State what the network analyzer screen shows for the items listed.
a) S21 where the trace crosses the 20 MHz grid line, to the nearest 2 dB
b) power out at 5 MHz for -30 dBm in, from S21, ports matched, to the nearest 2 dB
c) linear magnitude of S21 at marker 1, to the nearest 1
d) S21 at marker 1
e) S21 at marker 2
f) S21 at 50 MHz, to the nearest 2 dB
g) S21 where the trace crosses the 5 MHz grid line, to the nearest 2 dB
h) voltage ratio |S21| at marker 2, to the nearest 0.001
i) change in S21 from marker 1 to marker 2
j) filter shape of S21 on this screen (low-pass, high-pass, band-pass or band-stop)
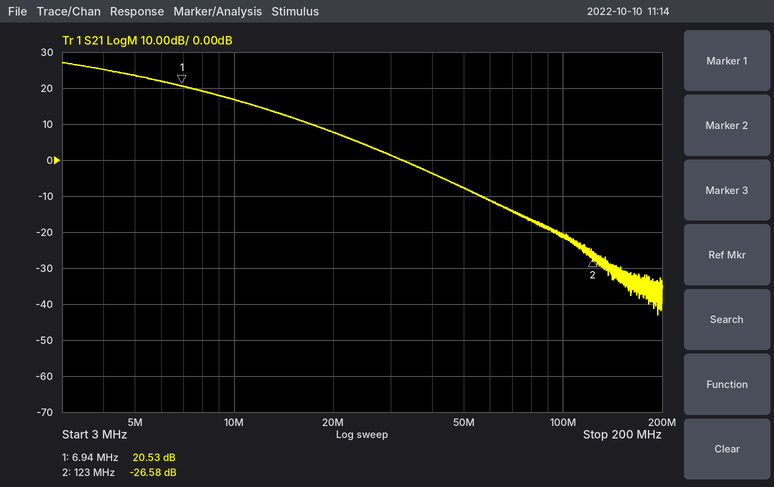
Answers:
8 dB
-6 dBm
11
20.53 dB
-26.58 dB
-8 dB
24 dB
0.047
-47.11 dB
low-pass
